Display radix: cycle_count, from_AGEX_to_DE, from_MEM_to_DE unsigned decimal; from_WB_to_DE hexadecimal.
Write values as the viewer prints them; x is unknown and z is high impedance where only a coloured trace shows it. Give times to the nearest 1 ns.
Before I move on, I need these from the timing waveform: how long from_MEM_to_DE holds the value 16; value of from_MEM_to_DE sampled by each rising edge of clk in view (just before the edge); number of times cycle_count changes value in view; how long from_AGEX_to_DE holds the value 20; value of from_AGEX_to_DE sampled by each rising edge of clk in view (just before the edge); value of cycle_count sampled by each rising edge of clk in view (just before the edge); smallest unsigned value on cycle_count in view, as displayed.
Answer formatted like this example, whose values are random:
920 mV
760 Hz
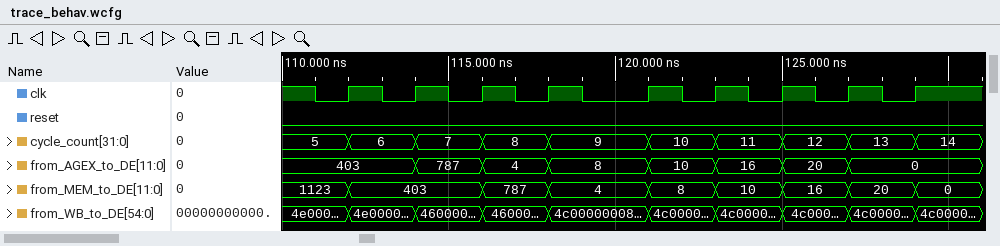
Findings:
2 ns
1123, 403, 403, 787, 4, 8, 10, 16, 20
9
2 ns
403, 403, 787, 4, 8, 10, 16, 20, 0
5, 6, 7, 8, 9, 10, 11, 12, 13
5
